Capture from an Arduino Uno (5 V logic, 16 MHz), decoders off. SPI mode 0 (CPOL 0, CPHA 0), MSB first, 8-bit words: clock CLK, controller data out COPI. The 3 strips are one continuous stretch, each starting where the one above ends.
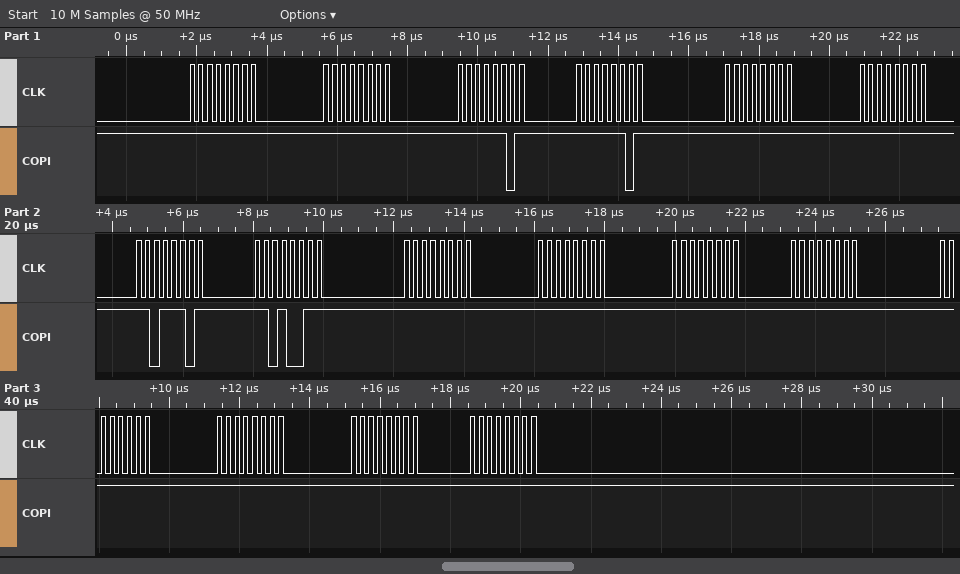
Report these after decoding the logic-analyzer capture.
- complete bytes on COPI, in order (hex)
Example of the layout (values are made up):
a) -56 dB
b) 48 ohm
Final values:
a) 0xFF 0xFF 0xFD 0xFD 0xFF 0xFF 0xDD 0xD3 0xFF 0xFF 0xFF 0xFF 0xFF 0xFF 0xFF 0xFF
